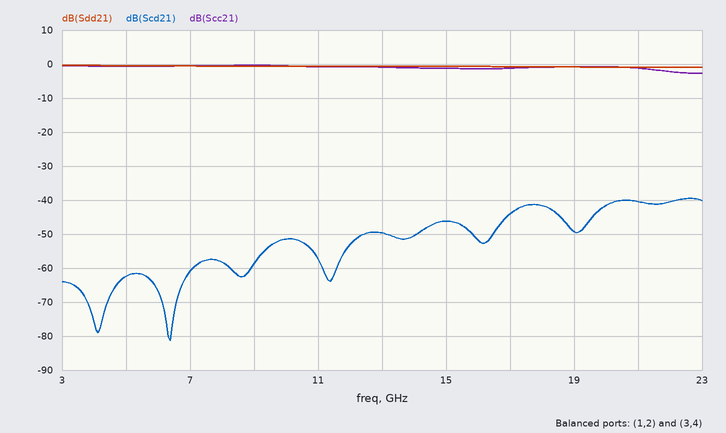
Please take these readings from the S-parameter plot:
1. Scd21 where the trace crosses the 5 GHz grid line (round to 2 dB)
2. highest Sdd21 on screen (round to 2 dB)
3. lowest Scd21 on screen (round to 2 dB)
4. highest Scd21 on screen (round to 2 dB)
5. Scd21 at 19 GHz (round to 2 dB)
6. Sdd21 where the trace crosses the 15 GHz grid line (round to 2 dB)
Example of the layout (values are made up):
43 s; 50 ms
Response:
-62 dB; 0 dB; -82 dB; -40 dB; -50 dB; 0 dB
